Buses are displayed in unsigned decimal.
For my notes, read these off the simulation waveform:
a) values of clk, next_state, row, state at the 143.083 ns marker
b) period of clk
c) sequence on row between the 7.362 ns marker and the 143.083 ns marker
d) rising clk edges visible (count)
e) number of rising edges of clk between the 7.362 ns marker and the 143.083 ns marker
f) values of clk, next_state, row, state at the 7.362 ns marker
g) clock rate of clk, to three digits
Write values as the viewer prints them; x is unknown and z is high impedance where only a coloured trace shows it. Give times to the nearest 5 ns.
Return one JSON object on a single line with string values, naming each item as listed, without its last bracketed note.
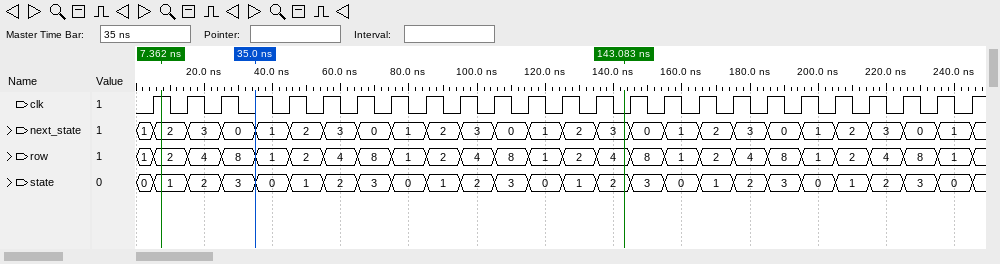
{"values of clk, next_state, row, state at the 143.083 ns marker": "clk=0, next_state=3, row=4, state=2", "period of clk": "10 ns", "sequence on row between the 7.362 ns marker and the 143.083 ns marker": "2, 4, 8, 1, 2, 4, 8, 1, 2, 4, 8, 1, 2, 4", "rising clk edges visible": "25", "number of rising edges of clk between the 7.362 ns marker and the 143.083 ns marker": "13", "values of clk, next_state, row, state at the 7.362 ns marker": "clk=1, next_state=2, row=2, state=1", "clock rate of clk, to three digits": "100 MHz"}
